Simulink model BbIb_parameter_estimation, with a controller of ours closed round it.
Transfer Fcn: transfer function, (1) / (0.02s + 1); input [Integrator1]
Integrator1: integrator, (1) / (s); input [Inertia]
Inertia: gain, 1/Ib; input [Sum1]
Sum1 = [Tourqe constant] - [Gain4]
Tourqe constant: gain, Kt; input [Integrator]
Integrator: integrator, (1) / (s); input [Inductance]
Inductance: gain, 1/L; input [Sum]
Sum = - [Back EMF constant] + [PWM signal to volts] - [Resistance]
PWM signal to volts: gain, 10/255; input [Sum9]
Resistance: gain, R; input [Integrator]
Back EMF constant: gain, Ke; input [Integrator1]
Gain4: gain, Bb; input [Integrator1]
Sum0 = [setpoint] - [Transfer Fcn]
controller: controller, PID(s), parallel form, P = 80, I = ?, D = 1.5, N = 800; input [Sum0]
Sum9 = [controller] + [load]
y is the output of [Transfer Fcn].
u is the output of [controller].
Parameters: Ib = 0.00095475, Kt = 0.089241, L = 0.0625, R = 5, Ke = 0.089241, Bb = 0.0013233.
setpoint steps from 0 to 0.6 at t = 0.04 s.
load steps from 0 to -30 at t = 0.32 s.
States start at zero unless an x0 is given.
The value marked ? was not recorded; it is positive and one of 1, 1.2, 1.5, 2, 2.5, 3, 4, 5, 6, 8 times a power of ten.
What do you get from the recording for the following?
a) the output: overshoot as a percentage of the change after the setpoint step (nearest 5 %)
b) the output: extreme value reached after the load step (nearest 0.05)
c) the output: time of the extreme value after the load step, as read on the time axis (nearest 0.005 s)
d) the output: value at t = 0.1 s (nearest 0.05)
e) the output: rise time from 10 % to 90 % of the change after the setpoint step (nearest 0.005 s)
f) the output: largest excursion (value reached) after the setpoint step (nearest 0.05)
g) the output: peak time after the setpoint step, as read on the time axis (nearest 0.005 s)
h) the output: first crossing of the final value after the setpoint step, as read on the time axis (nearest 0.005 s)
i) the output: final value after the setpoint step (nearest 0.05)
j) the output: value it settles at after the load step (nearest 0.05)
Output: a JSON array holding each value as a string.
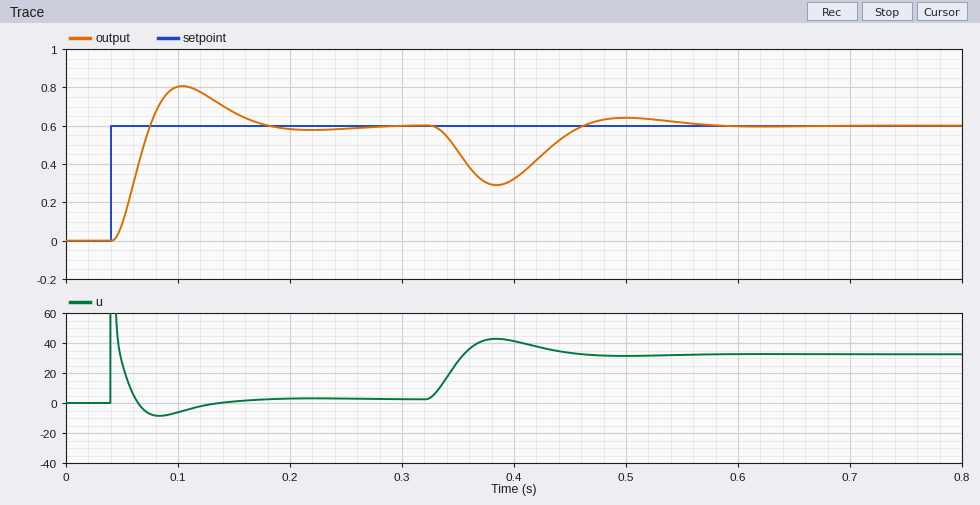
["35 %", "0.30", "0.385 s", "0.80", "0.025 s", "0.80", "0.105 s", "0.075 s", "0.60", "0.60"]
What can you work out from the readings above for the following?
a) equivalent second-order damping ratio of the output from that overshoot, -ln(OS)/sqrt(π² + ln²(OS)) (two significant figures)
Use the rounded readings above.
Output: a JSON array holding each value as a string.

["0.32"]
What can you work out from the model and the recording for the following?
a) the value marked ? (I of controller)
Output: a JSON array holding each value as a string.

["1500"]
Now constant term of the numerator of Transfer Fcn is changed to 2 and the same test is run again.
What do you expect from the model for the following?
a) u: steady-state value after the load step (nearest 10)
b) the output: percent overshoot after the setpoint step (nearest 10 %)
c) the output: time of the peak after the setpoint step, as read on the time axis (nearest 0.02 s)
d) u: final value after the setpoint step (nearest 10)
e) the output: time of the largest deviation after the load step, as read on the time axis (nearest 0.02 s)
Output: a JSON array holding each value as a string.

["30", "40 %", "0.08 s", "0", "0.36 s"]
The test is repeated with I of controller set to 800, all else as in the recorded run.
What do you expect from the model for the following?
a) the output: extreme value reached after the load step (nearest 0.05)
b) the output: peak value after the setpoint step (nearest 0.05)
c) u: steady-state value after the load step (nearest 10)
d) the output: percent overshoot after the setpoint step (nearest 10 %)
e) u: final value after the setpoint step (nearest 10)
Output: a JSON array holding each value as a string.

["0.25", "0.75", "30", "20 %", "0"]
